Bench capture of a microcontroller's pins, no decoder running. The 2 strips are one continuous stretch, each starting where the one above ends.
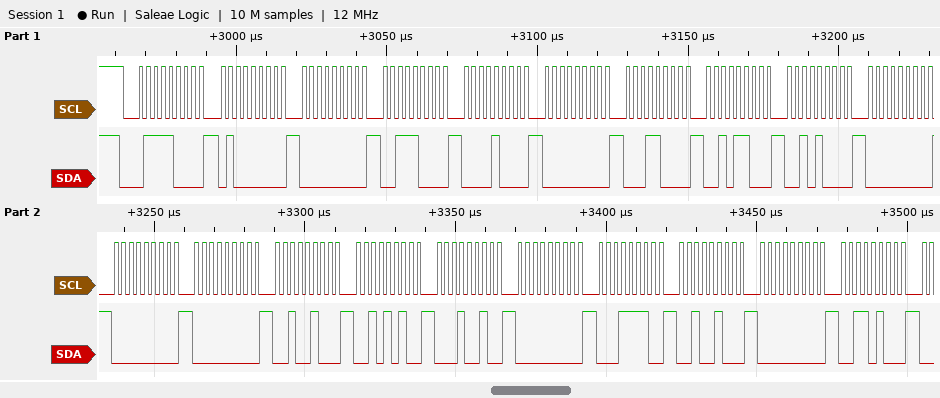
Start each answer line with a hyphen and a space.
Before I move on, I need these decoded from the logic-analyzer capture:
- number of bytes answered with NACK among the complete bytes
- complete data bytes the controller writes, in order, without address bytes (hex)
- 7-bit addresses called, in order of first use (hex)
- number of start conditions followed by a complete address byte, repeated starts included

- 0
- 40 00 38 08 00 18 2C 28 00 00 00 24 2A 12 00 1E 24 00 34
- 0x3C
- 1
